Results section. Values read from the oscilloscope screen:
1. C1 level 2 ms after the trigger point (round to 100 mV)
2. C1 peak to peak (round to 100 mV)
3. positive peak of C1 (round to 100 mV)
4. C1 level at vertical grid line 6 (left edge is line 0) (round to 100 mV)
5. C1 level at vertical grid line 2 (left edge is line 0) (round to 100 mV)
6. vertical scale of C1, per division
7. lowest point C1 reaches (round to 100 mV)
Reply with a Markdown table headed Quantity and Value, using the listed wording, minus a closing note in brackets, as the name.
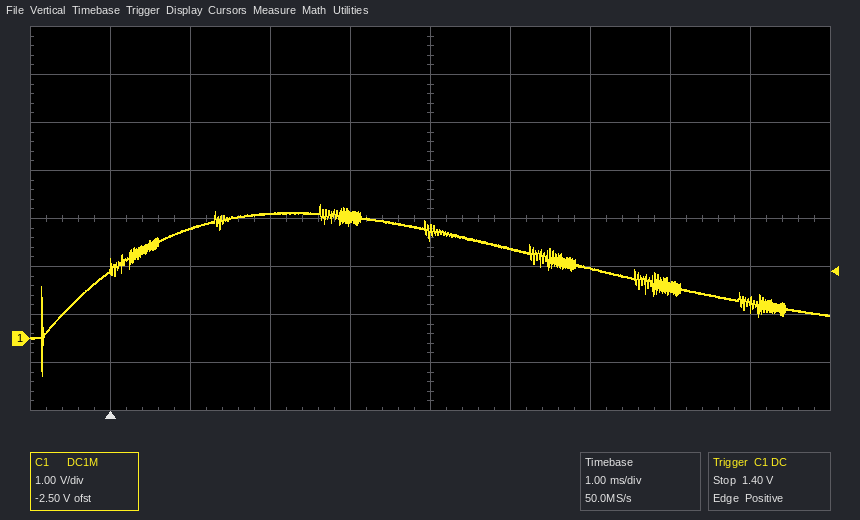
| Quantity | Value |
|---|---|
| C1 level 2 ms after the trigger point | 2.6 V |
| C1 peak to peak | 3.6 V |
| positive peak of C1 | 2.8 V |
| C1 level at vertical grid line 6 (left edge is line 0) | 1.9 V |
| C1 level at vertical grid line 2 (left edge is line 0) | 2.3 V |
| vertical scale of C1, per division | 1 V |
| lowest point C1 reaches | -800 mV |
